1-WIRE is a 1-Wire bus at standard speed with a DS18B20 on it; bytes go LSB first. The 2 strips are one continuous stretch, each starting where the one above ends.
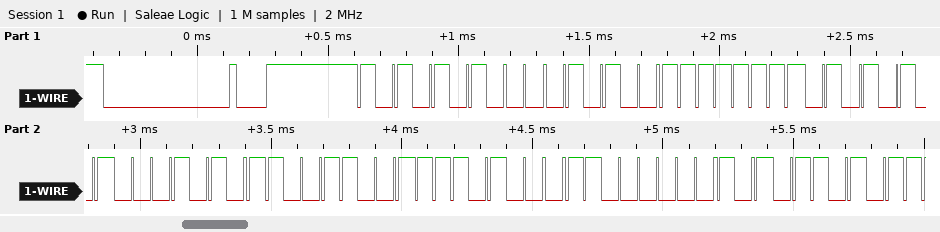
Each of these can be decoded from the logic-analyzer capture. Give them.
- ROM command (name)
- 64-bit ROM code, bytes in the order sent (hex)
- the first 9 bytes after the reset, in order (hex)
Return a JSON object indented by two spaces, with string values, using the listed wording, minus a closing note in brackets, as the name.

{
  "ROM command": "Match ROM",
  "64-bit ROM code, bytes in the order sent": "28 FF AA A8 99 17 03 B5",
  "the first 9 bytes after the reset, in order": "55 28 FF AA A8 99 17 03 B5"
}
